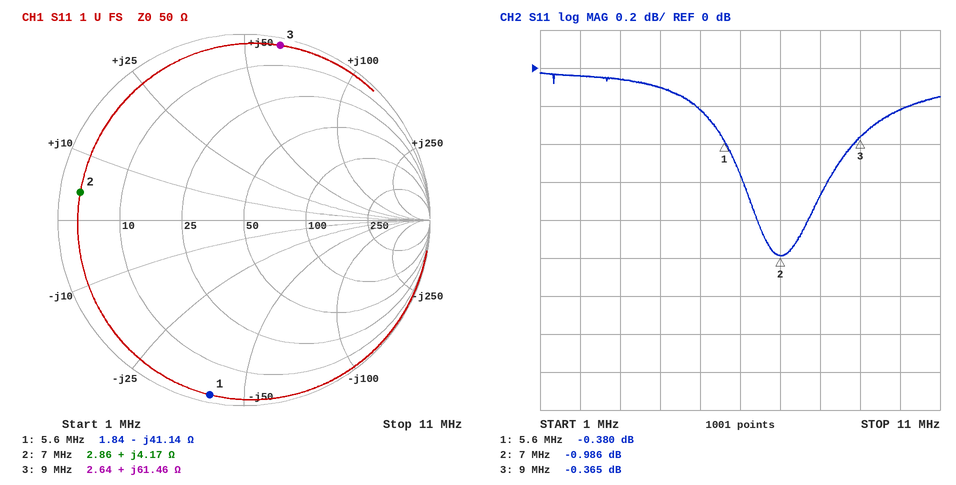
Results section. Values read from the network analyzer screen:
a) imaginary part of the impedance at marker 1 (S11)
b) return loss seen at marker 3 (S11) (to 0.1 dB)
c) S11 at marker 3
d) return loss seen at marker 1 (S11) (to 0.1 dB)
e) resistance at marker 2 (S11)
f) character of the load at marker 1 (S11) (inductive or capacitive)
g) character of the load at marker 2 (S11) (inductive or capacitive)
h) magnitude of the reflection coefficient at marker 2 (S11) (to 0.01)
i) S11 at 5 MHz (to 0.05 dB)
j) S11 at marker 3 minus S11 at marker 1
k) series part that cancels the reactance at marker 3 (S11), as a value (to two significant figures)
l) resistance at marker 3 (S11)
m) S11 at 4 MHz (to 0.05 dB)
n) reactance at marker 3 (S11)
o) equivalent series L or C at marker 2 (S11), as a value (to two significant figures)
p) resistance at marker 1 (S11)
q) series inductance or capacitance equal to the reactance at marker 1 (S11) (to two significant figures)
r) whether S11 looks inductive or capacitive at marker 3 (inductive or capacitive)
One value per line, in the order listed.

-41.14 Ω
0.4 dB
-0.365 dB
0.4 dB
2.86 Ω
capacitive
inductive
0.89
-0.20 dB
0.015 dB
290 pF
2.64 Ω
-0.10 dB
+61.46 Ω
95 nH
1.84 Ω
690 pF
inductive
